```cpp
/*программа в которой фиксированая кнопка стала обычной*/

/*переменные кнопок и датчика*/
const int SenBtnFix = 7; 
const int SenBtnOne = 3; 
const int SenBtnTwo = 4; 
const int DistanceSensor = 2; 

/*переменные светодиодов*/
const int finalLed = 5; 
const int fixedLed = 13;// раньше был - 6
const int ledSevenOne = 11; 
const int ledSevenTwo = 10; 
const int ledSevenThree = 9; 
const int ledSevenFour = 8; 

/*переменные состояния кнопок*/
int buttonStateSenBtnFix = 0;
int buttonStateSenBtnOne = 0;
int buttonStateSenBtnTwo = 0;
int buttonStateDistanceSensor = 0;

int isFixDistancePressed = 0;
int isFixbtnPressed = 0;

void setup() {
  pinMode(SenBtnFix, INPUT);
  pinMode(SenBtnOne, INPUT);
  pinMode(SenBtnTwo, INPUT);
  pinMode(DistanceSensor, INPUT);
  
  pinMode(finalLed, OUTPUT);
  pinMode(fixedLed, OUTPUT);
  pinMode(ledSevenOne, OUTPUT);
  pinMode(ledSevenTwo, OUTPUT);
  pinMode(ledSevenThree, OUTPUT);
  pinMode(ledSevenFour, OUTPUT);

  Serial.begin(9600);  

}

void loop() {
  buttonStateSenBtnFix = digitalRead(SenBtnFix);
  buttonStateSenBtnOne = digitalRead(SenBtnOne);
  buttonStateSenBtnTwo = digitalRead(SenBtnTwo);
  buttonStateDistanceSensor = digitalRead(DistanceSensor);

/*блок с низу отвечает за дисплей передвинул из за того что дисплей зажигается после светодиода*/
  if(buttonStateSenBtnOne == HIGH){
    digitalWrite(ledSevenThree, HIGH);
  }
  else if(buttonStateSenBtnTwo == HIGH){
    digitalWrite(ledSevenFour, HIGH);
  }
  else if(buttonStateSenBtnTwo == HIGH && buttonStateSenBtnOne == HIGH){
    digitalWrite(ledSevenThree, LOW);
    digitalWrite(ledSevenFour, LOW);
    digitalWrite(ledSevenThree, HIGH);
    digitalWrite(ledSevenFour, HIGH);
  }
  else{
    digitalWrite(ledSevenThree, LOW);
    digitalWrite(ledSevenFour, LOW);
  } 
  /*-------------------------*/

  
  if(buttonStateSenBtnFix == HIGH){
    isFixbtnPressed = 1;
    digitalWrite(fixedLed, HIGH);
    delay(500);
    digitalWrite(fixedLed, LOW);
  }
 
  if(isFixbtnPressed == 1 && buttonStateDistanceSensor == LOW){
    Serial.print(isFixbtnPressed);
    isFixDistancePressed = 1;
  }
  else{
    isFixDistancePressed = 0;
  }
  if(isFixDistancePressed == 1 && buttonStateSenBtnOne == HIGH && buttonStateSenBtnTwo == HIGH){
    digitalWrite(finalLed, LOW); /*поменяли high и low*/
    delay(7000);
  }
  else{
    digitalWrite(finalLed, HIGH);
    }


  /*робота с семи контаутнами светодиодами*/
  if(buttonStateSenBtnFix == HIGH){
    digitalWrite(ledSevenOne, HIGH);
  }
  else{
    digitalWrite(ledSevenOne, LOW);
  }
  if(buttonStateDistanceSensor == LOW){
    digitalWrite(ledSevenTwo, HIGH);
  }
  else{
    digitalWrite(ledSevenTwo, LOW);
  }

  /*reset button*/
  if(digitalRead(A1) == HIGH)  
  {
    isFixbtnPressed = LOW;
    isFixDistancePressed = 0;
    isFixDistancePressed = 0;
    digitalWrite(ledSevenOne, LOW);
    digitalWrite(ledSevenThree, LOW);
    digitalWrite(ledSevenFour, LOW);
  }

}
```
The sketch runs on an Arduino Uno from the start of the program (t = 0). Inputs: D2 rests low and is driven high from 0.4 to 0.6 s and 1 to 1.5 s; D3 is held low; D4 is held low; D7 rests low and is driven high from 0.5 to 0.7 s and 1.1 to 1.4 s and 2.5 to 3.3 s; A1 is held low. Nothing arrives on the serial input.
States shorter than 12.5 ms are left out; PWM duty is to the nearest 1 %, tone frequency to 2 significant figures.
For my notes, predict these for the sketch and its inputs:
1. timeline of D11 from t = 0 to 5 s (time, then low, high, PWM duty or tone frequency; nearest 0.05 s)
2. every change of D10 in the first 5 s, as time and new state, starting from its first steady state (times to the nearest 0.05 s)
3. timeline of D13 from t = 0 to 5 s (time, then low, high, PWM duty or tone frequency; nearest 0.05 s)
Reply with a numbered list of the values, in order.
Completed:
1. 0 s low; 3 s high; 3.5 s low
2. 0 s high; 0.4 s low; 1.6 s high
3. 0 s low; 0.5 s high; 1 s low; 1.1 s high; 1.6 s low; 2.5 s high; 3.5 s low
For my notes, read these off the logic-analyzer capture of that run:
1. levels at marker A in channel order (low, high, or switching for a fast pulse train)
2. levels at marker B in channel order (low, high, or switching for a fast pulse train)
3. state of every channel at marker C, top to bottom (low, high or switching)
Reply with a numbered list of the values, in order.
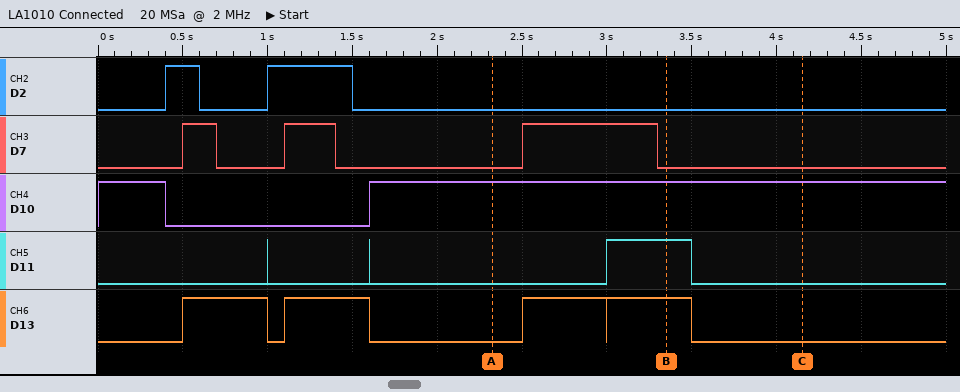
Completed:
1. D2 low, D7 low, D10 high, D11 low, D13 low
2. D2 low, D7 low, D10 high, D11 high, D13 high
3. D2 low, D7 low, D10 high, D11 low, D13 low
